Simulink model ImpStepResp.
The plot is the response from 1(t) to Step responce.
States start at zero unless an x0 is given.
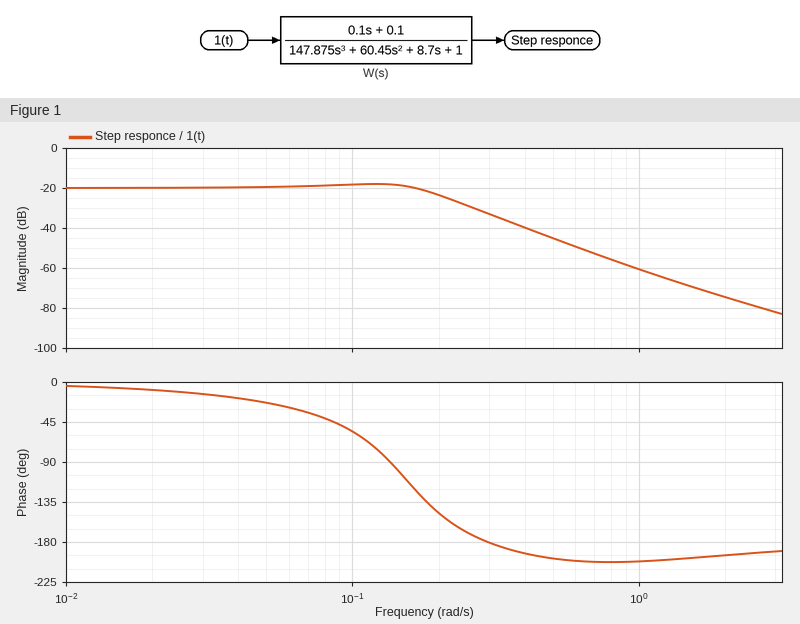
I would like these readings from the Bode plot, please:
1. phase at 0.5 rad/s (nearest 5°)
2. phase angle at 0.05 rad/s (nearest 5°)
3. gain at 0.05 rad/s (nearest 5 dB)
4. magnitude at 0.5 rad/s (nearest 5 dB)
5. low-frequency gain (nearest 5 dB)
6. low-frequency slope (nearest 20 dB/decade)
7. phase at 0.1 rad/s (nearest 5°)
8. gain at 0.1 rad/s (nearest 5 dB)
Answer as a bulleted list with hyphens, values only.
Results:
- -200°
- -25°
- -20 dB
- -45 dB
- -20 dB
- 0 dB/decade
- -55°
- -20 dB
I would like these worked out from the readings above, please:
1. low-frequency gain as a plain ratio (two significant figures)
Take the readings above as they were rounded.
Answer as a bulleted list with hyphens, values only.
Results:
- 0.10
